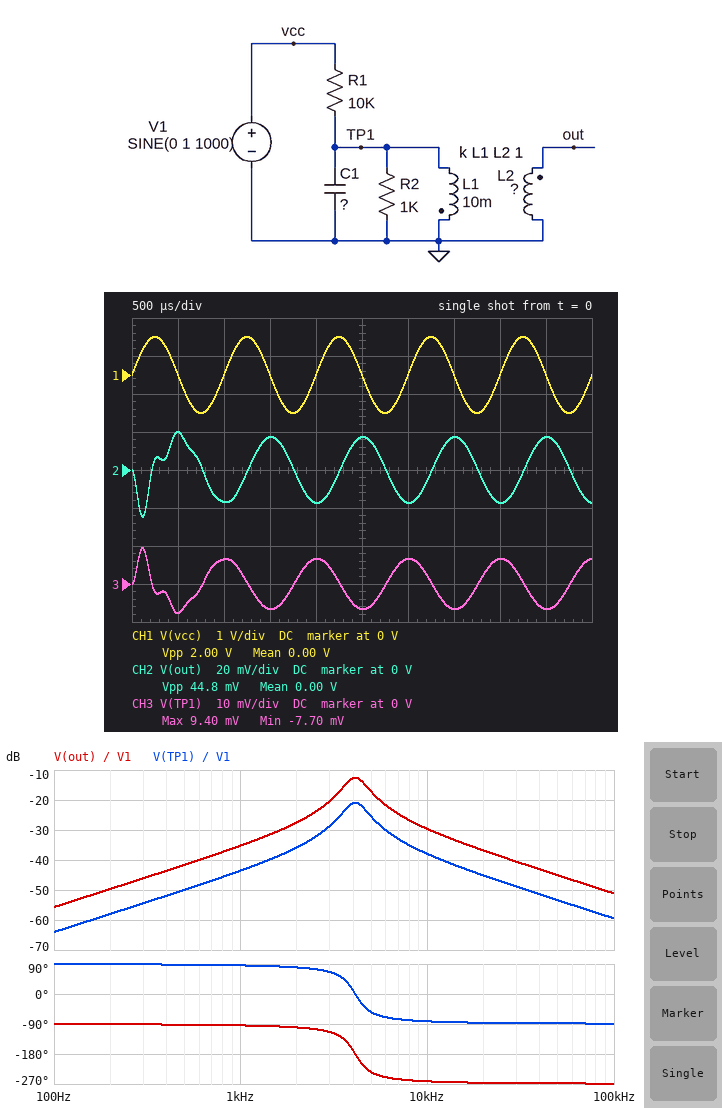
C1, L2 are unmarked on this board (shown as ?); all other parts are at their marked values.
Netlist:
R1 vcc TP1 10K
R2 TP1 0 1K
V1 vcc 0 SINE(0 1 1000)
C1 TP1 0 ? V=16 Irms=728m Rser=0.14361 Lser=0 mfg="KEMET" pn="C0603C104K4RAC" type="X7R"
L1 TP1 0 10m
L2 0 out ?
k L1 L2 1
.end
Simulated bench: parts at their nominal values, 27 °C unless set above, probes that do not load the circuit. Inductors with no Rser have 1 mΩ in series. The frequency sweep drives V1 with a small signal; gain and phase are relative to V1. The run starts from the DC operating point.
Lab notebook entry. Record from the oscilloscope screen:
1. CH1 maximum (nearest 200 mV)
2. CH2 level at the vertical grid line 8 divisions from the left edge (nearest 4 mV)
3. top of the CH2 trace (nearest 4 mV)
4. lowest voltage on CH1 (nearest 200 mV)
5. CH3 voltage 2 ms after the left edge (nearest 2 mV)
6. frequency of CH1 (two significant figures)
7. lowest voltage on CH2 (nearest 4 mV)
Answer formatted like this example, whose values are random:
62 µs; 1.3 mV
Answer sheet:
1.0 V; -16 mV; 20 mV; -1.0 V; 6 mV; 1.0 kHz; -24 mV
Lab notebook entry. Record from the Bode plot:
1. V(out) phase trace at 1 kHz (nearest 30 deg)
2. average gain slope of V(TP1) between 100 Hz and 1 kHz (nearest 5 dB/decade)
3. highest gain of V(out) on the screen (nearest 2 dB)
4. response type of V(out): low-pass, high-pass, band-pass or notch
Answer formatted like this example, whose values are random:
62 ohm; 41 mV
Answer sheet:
-90 deg; 20 dB/decade; -12 dB; band-pass
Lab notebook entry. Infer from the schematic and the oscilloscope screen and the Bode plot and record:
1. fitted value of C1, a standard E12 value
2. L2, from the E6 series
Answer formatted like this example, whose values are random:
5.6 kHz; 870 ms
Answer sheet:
150 nF; 68 mH
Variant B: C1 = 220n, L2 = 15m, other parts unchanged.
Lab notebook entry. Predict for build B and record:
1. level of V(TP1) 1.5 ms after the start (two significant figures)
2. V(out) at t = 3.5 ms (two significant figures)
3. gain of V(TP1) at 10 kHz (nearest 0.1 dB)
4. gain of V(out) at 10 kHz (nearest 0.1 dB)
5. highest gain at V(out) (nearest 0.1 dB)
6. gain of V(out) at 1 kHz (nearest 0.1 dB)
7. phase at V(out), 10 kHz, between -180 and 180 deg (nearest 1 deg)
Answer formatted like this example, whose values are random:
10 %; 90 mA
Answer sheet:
-7.0 mV; 8.4 mV; -41.8 dB; -40.0 dB; -19.1 dB; -41.5 dB; 95 deg
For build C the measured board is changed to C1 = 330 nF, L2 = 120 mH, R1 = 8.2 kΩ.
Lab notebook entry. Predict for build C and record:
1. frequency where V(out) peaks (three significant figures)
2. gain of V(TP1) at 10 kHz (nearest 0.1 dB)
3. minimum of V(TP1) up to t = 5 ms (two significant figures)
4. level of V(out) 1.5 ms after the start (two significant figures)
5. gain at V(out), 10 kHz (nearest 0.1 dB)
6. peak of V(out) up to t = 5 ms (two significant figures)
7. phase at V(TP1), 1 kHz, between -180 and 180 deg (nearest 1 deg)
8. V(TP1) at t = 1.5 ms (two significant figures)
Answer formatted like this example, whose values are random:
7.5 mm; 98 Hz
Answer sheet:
2.77 kHz; -43.9 dB; -11 mV; 32 mV; -33.1 dB; 37 mV; 85 deg; -9.3 mV
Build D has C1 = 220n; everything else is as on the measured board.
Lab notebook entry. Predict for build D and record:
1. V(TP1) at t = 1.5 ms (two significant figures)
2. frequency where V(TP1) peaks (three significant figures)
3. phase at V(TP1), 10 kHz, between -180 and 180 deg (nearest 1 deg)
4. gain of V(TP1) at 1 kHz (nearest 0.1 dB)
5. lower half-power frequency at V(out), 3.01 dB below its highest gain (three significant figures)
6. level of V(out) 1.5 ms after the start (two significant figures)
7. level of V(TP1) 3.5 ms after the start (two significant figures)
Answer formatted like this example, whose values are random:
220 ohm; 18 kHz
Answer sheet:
-7.0 mV; 3.39 kHz; -85 deg; -43.3 dB; 3.02 kHz; 18 mV; -6.8 mV
